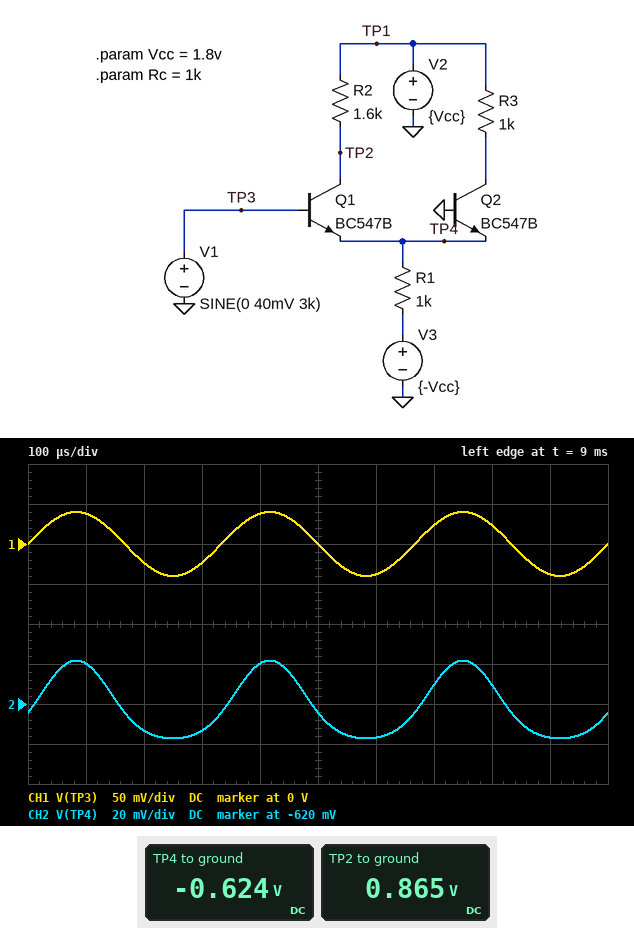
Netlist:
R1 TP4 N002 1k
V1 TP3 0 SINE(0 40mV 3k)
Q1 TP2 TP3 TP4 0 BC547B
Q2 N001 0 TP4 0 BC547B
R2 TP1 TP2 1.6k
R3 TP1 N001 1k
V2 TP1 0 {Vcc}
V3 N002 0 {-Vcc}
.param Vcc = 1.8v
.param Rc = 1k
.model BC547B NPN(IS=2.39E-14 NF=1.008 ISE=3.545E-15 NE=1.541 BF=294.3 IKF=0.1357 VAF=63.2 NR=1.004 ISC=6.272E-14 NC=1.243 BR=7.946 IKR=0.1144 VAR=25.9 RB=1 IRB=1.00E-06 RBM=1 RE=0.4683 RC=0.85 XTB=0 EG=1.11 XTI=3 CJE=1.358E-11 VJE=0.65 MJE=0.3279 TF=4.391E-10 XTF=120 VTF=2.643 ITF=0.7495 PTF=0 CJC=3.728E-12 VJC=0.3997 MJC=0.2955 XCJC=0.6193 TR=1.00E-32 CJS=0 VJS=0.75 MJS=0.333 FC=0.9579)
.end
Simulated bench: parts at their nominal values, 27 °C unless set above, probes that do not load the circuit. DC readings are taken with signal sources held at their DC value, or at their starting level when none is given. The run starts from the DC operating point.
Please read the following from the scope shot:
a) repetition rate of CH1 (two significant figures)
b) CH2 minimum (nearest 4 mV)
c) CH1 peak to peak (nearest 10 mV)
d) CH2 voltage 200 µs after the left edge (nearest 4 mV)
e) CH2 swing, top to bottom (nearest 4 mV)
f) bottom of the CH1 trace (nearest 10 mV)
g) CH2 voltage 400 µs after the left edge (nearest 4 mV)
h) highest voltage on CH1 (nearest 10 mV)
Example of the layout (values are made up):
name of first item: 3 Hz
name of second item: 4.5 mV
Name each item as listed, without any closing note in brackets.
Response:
repetition rate of CH1: 3.0 kHz
CH2 minimum: -636 mV
CH1 peak to peak: 80 mV
CH2 voltage 200 µs after the left edge: -632 mV
CH2 swing, top to bottom: 40 mV
bottom of the CH1 trace: -40 mV
CH2 voltage 400 µs after the left edge: -600 mV
highest voltage on CH1: 40 mV
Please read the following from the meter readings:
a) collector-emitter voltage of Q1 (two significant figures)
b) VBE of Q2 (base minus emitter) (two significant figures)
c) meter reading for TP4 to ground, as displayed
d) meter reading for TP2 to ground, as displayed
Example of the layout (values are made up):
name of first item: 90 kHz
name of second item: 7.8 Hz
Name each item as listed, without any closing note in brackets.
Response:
collector-emitter voltage of Q1: 1.5 V
VBE of Q2 (base minus emitter): 620 mV
meter reading for TP4 to ground, as displayed: -0.624 V
meter reading for TP2 to ground, as displayed: 0.865 V
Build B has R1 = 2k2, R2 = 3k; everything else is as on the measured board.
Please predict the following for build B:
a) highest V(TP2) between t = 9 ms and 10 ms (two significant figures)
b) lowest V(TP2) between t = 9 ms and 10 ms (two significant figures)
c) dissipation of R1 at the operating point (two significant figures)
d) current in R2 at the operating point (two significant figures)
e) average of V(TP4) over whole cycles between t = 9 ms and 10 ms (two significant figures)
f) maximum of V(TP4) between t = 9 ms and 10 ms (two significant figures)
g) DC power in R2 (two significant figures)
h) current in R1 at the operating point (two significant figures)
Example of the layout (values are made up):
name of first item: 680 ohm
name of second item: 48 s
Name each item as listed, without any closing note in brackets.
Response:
highest V(TP2) between t = 9 ms and 10 ms: 1.5 V
lowest V(TP2) between t = 9 ms and 10 ms: 440 mV
dissipation of R1 at the operating point: 650 µW
current in R2 at the operating point: 270 µA
average of V(TP4) over whole cycles between t = 9 ms and 10 ms: -600 mV
maximum of V(TP4) between t = 9 ms and 10 ms: -580 mV
DC power in R2: 220 µW
current in R1 at the operating point: 540 µA
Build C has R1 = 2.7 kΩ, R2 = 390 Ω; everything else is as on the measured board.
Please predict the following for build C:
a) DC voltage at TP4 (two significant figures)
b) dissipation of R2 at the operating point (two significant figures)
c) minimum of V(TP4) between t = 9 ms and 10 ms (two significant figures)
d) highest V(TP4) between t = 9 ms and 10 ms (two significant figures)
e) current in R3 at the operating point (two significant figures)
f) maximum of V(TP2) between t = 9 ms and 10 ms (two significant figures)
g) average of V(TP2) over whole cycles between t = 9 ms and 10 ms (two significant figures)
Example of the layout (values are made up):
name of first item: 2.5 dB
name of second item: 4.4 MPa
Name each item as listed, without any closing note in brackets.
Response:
DC voltage at TP4: -600 mV
dissipation of R2 at the operating point: 19 µW
minimum of V(TP4) between t = 9 ms and 10 ms: -610 mV
highest V(TP4) between t = 9 ms and 10 ms: -570 mV
current in R3 at the operating point: 220 µA
maximum of V(TP2) between t = 9 ms and 10 ms: 1.8 V
average of V(TP2) over whole cycles between t = 9 ms and 10 ms: 1.7 V
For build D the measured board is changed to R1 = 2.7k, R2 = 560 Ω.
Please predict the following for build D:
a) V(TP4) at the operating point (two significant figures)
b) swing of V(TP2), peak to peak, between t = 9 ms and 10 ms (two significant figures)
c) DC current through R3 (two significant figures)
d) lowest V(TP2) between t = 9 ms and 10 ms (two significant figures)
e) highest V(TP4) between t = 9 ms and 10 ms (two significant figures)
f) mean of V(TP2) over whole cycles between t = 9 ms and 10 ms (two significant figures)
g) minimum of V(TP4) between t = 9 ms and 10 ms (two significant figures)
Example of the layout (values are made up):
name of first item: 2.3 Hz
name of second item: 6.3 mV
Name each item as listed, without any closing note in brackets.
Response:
V(TP4) at the operating point: -600 mV
swing of V(TP2), peak to peak, between t = 9 ms and 10 ms: 160 mV
DC current through R3: 220 µA
lowest V(TP2) between t = 9 ms and 10 ms: 1.6 V
highest V(TP4) between t = 9 ms and 10 ms: -570 mV
mean of V(TP2) over whole cycles between t = 9 ms and 10 ms: 1.7 V
minimum of V(TP4) between t = 9 ms and 10 ms: -610 mV
